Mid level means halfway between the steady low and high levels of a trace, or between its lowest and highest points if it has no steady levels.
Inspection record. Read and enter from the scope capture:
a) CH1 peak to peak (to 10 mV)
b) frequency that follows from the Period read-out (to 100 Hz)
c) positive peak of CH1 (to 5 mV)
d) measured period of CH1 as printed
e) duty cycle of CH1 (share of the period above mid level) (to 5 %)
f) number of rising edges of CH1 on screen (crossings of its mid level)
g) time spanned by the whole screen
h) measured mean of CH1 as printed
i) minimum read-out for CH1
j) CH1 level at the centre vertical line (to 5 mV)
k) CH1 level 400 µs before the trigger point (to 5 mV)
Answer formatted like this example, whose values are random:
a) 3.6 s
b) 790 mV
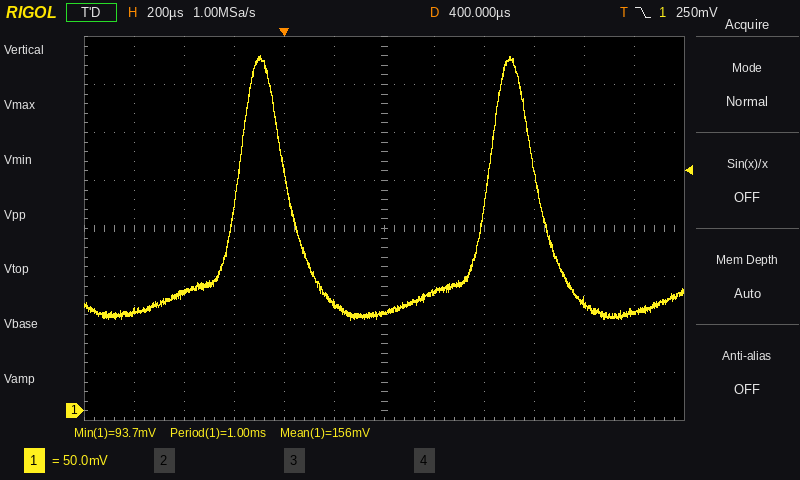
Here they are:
a) 280 mV
b) 1.0 kHz
c) 370 mV
d) 1.00 ms
e) 20 %
f) 2
g) 2.4 ms
h) 156 mV
i) 93.7 mV
j) 100 mV
k) 125 mV
